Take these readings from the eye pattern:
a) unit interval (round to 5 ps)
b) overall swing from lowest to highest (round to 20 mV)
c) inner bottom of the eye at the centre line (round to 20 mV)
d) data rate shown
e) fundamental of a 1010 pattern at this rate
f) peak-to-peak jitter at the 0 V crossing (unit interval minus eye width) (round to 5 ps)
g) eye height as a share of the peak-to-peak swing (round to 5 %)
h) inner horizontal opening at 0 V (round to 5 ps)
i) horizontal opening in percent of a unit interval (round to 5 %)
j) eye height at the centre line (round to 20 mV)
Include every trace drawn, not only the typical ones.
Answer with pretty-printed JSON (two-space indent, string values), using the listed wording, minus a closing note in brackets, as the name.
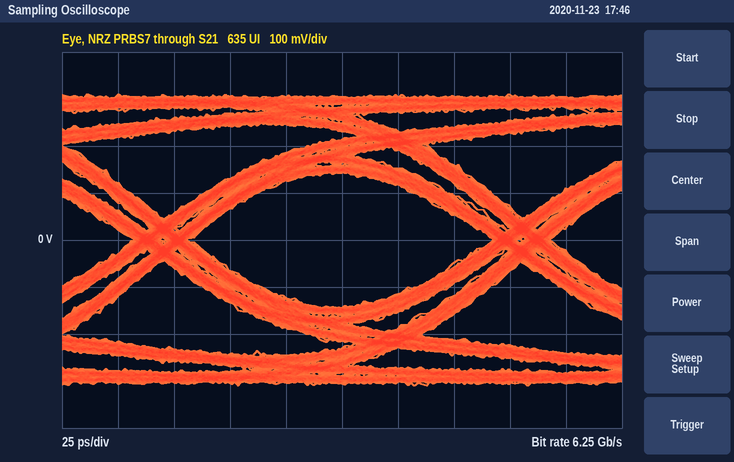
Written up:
{
  "unit interval": "160 ps",
  "overall swing from lowest to highest": "620 mV",
  "inner bottom of the eye at the centre line": "-140 mV",
  "data rate shown": "6.25 Gb/s",
  "fundamental of a 1010 pattern at this rate": "3.125 GHz",
  "peak-to-peak jitter at the 0 V crossing (unit interval minus eye width)": "25 ps",
  "eye height as a share of the peak-to-peak swing": "45 %",
  "inner horizontal opening at 0 V": "135 ps",
  "horizontal opening in percent of a unit interval": "85 %",
  "eye height at the centre line": "280 mV"
}
